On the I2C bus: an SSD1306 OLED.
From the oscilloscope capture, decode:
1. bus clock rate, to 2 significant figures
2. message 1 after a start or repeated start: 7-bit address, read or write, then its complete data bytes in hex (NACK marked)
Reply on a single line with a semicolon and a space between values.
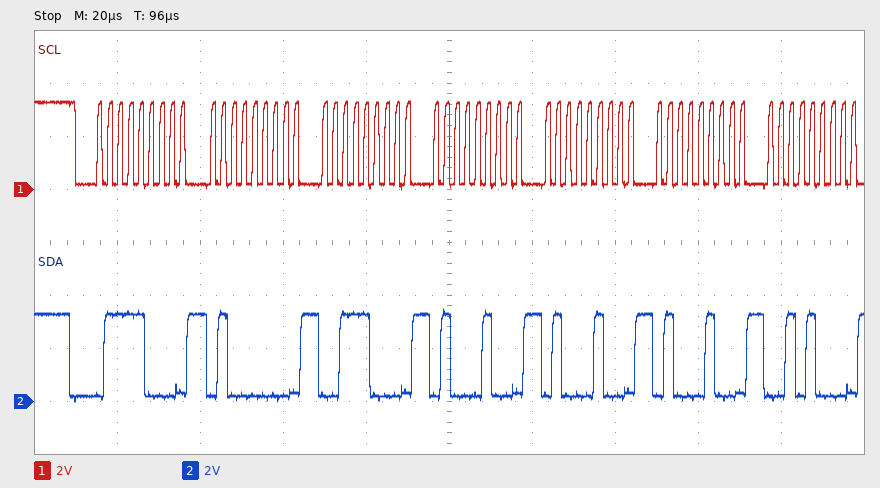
400 kHz; 0x3C write: 40 38 44 44 44 28
